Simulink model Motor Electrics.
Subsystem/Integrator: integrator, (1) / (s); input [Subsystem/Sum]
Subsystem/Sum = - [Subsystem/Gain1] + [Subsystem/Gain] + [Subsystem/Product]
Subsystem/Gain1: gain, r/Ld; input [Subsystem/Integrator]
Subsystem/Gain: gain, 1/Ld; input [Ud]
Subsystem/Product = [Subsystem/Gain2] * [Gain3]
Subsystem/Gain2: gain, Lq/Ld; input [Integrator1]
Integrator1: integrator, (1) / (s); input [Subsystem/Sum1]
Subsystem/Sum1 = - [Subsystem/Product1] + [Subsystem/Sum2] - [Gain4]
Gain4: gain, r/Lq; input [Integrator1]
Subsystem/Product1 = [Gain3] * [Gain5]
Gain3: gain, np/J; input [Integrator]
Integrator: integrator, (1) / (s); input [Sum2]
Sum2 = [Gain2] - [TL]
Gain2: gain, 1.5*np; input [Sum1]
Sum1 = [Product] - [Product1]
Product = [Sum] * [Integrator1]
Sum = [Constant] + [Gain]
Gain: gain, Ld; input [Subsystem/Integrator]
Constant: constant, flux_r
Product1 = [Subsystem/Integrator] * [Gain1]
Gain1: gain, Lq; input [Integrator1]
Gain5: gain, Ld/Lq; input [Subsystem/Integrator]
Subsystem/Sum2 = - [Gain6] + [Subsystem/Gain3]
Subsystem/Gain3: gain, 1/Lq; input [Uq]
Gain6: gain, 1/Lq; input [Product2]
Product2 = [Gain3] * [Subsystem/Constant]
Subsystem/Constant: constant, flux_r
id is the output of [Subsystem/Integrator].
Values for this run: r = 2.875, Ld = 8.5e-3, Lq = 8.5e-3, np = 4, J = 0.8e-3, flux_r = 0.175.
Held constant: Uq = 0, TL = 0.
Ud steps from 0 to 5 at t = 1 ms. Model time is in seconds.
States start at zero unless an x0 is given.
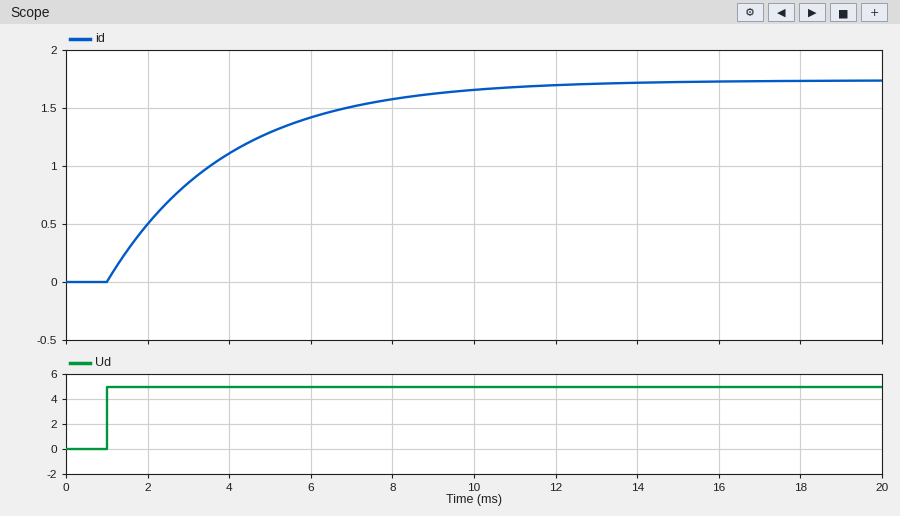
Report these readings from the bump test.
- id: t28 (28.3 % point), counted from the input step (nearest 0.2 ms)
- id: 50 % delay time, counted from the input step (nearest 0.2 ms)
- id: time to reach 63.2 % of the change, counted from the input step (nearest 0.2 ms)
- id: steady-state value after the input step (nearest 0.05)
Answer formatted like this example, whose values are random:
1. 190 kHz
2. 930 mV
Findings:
1. 1.0 ms
2. 2.0 ms
3. 3.0 ms
4. 1.75
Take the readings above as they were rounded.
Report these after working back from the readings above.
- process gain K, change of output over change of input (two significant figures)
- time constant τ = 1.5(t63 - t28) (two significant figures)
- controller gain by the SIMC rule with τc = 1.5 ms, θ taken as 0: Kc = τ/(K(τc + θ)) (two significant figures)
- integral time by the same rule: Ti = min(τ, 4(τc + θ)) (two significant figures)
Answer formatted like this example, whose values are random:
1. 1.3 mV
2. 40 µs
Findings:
1. 0.35
2. 3.0 ms
3. 5.7
4. 3.0 ms
